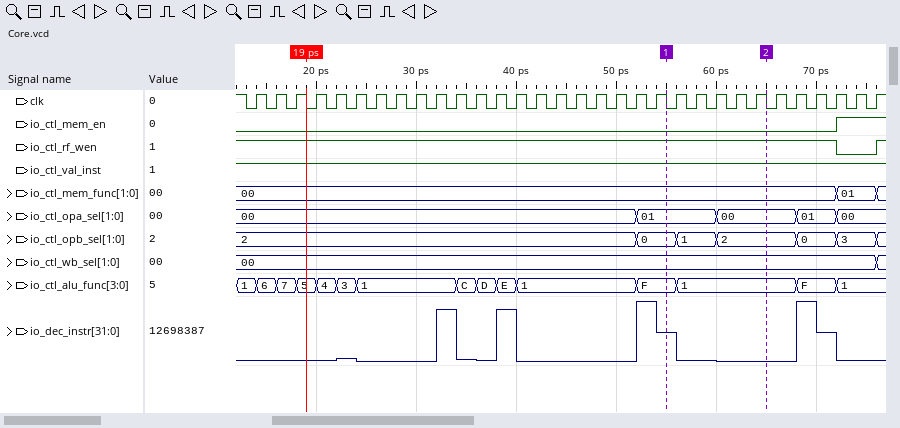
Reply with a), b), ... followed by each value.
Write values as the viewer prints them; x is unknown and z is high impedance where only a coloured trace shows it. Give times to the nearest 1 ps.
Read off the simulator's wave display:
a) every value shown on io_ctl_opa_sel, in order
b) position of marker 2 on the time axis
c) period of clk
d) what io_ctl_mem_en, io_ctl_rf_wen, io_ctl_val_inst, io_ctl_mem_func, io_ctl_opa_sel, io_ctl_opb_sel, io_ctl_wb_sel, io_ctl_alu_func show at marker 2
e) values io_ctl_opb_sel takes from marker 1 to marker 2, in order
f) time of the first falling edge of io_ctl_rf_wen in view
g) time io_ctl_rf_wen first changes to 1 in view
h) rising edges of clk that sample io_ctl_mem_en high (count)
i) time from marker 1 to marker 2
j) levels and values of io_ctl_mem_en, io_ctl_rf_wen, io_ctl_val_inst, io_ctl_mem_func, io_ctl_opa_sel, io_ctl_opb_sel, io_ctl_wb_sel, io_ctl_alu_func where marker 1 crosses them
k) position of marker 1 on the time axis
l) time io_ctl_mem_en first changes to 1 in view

a) 00, 01, 00, 01, 00
b) 65 ps
c) 2 ps
d) io_ctl_mem_en=0, io_ctl_rf_wen=1, io_ctl_val_inst=1, io_ctl_mem_func=00, io_ctl_opa_sel=00, io_ctl_opb_sel=2, io_ctl_wb_sel=00, io_ctl_alu_func=1
e) 0, 1, 2
f) 72 ps
g) 76 ps
h) 2
i) 10 ps
j) io_ctl_mem_en=0, io_ctl_rf_wen=1, io_ctl_val_inst=1, io_ctl_mem_func=00, io_ctl_opa_sel=01, io_ctl_opb_sel=0, io_ctl_wb_sel=00, io_ctl_alu_func=F
k) 55 ps
l) 72 ps
